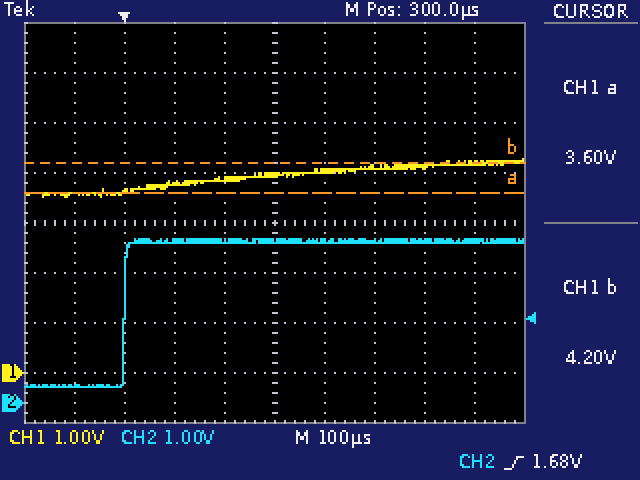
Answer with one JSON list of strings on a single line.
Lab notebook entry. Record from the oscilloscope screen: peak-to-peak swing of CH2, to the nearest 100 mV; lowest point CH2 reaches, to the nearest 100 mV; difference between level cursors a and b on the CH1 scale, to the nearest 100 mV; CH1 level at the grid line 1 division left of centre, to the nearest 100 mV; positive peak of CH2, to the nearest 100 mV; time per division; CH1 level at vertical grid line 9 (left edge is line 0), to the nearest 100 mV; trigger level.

["3.0 V", "300 mV", "600 mV", "3.9 V", "3.3 V", "100 µs", "4.2 V", "1.68 V"]
